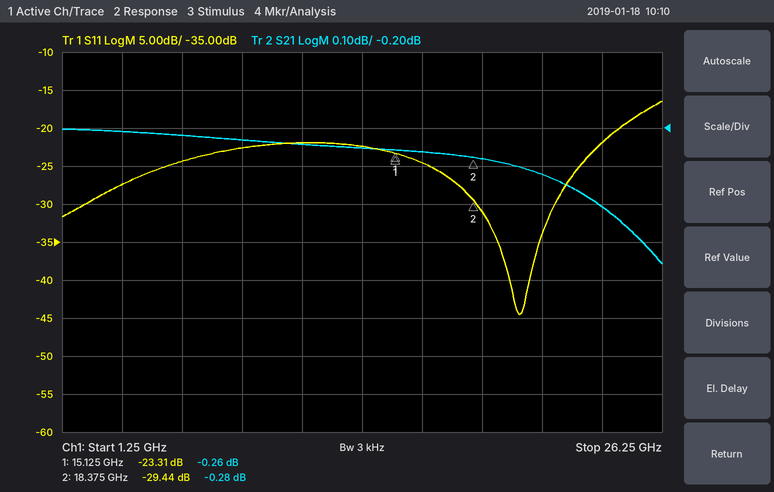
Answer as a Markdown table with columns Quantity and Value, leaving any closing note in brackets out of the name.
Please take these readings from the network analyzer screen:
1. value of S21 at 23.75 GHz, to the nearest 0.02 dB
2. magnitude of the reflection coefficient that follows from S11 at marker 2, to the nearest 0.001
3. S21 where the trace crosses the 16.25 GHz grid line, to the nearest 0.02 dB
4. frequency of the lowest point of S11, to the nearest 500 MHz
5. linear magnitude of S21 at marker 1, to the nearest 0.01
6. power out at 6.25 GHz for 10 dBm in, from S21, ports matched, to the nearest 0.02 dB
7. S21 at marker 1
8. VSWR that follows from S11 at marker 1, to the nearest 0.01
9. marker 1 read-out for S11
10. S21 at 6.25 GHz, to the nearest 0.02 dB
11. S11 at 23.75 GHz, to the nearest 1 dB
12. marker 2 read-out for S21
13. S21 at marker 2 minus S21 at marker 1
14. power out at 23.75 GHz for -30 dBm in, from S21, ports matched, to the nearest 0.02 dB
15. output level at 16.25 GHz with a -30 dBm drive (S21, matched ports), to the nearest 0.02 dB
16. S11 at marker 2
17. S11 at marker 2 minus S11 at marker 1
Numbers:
| Quantity | Value |
|---|---|
| value of S21 at 23.75 GHz, to the nearest 0.02 dB | -0.40 dB |
| magnitude of the reflection coefficient that follows from S11 at marker 2, to the nearest 0.001 | 0.034 |
| S21 where the trace crosses the 16.25 GHz grid line, to the nearest 0.02 dB | -0.26 dB |
| frequency of the lowest point of S11, to the nearest 500 MHz | 20.5 GHz |
| linear magnitude of S21 at marker 1, to the nearest 0.01 | 0.97 |
| power out at 6.25 GHz for 10 dBm in, from S21, ports matched, to the nearest 0.02 dB | 9.78 dBm |
| S21 at marker 1 | -0.26 dB |
| VSWR that follows from S11 at marker 1, to the nearest 0.01 | 1.15 |
| marker 1 read-out for S11 | -23.31 dB |
| S21 at 6.25 GHz, to the nearest 0.02 dB | -0.22 dB |
| S11 at 23.75 GHz, to the nearest 1 dB | -22 dB |
| marker 2 read-out for S21 | -0.28 dB |
| S21 at marker 2 minus S21 at marker 1 | -0.02 dB |
| power out at 23.75 GHz for -30 dBm in, from S21, ports matched, to the nearest 0.02 dB | -30.40 dBm |
| output level at 16.25 GHz with a -30 dBm drive (S21, matched ports), to the nearest 0.02 dB | -30.26 dBm |
| S11 at marker 2 | -29.44 dB |
| S11 at marker 2 minus S11 at marker 1 | -6.13 dB |
